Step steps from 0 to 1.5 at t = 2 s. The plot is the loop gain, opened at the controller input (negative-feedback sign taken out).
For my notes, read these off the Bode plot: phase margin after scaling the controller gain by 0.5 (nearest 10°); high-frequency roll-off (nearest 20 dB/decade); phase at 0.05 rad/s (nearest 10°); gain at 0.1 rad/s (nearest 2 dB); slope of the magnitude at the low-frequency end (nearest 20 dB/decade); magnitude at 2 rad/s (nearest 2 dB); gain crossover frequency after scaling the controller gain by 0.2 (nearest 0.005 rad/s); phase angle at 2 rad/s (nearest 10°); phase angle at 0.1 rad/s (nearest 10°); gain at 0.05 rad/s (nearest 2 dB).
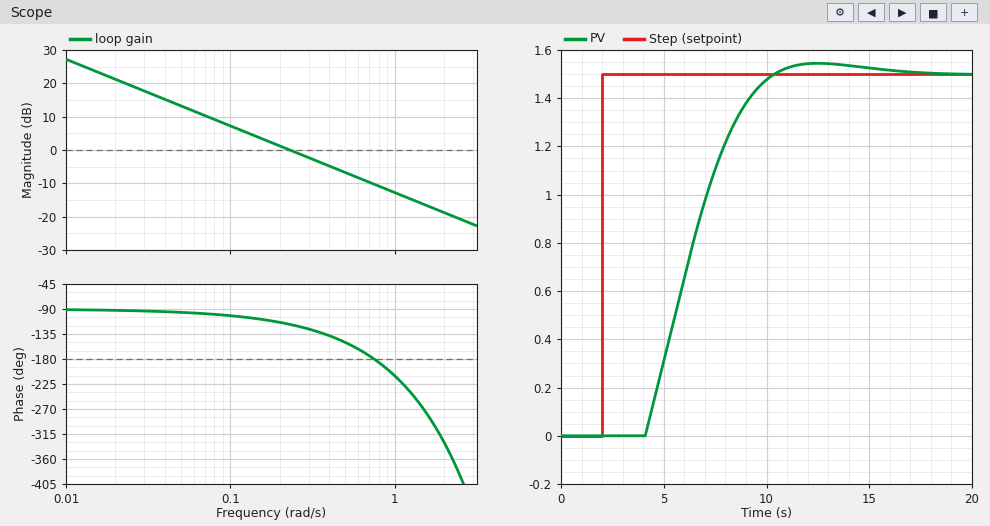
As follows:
80°
-20 dB/decade
-100°
8 dB
-20 dB/decade
-18 dB
0.045 rad/s
-330°
-100°
14 dB
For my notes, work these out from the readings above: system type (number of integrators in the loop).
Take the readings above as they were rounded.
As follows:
1
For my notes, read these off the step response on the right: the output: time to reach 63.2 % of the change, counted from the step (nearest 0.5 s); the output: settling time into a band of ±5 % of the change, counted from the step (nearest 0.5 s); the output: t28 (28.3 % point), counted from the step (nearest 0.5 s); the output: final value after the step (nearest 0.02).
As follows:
5.0 s
7.5 s
3.5 s
1.50
